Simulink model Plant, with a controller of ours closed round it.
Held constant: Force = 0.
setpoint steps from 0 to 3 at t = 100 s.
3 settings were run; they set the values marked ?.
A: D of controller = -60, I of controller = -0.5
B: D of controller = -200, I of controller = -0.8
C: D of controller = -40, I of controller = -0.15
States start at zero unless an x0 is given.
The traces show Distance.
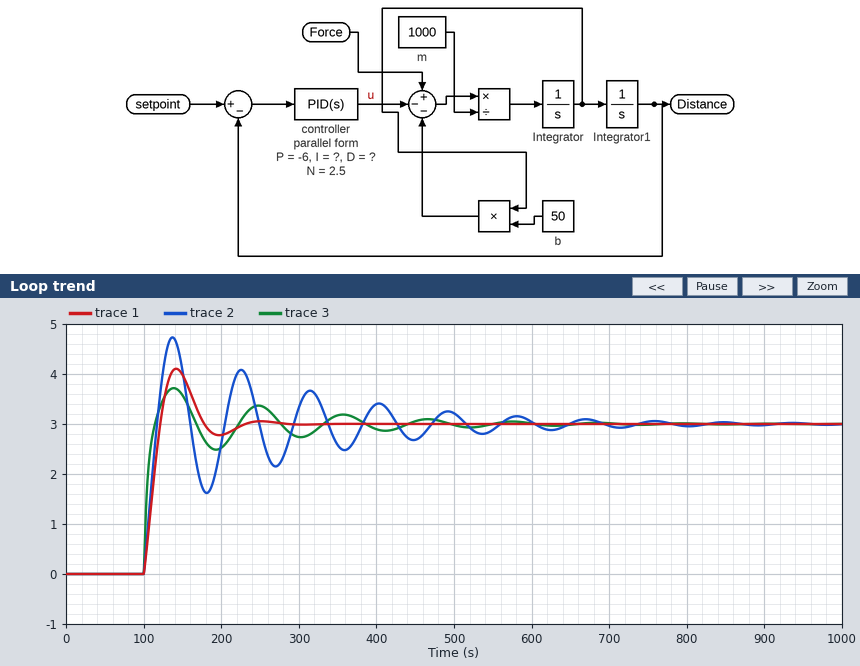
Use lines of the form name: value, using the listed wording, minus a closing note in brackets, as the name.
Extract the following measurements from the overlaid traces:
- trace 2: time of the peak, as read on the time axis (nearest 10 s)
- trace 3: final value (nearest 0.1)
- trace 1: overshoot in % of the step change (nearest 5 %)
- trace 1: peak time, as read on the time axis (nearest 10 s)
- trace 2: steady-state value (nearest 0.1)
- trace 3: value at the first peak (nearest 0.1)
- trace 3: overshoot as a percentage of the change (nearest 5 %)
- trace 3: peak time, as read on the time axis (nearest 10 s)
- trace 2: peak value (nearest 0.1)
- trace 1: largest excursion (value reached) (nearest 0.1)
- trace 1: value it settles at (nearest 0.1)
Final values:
trace 2: time of the peak, as read on the time axis: 140 s
trace 3: final value: 3.0
trace 1: overshoot in % of the step change: 35 %
trace 1: peak time, as read on the time axis: 140 s
trace 2: steady-state value: 3.0
trace 3: value at the first peak: 3.7
trace 3: overshoot as a percentage of the change: 25 %
trace 3: peak time, as read on the time axis: 140 s
trace 2: peak value: 4.7
trace 1: largest excursion (value reached): 4.1
trace 1: value it settles at: 3.0
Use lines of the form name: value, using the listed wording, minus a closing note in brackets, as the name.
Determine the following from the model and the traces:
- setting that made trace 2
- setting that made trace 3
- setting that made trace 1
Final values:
setting that made trace 2: A
setting that made trace 3: B
setting that made trace 1: C
